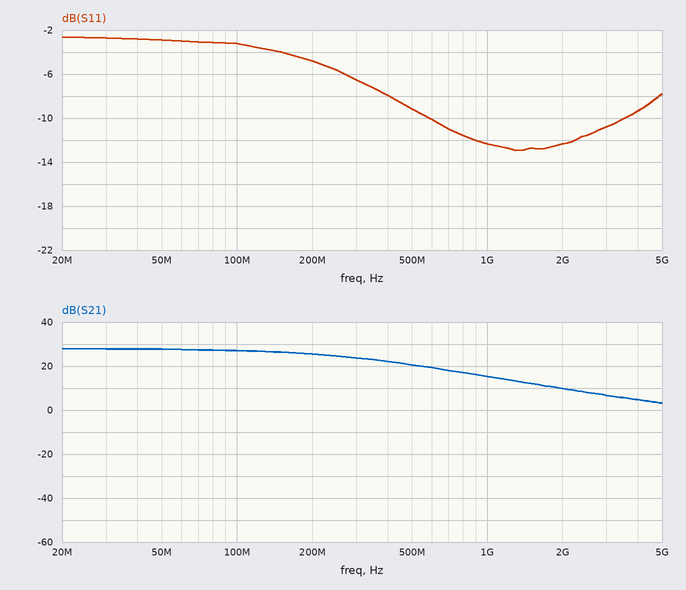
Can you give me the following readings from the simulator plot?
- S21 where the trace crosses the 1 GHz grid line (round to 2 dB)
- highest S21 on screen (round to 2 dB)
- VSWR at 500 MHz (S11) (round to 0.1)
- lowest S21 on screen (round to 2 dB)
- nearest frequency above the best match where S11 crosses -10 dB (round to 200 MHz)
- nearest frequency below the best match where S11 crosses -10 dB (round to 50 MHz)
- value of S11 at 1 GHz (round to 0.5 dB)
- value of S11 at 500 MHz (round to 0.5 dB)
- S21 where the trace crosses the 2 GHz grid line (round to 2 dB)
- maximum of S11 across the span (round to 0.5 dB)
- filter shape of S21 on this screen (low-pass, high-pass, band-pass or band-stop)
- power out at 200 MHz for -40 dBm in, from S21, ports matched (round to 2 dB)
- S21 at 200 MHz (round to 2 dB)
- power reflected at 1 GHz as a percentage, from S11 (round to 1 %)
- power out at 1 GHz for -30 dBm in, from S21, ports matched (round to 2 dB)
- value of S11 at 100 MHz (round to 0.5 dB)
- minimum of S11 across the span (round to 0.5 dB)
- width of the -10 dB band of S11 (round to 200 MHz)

16 dB
28 dB
2.1
4 dB
3.6 GHz
600 MHz
-12.5 dB
-9.0 dB
10 dB
-2.5 dB
low-pass
-14 dBm
26 dB
6 %
-14 dBm
-3.0 dB
-13.0 dB
3.0 GHz
